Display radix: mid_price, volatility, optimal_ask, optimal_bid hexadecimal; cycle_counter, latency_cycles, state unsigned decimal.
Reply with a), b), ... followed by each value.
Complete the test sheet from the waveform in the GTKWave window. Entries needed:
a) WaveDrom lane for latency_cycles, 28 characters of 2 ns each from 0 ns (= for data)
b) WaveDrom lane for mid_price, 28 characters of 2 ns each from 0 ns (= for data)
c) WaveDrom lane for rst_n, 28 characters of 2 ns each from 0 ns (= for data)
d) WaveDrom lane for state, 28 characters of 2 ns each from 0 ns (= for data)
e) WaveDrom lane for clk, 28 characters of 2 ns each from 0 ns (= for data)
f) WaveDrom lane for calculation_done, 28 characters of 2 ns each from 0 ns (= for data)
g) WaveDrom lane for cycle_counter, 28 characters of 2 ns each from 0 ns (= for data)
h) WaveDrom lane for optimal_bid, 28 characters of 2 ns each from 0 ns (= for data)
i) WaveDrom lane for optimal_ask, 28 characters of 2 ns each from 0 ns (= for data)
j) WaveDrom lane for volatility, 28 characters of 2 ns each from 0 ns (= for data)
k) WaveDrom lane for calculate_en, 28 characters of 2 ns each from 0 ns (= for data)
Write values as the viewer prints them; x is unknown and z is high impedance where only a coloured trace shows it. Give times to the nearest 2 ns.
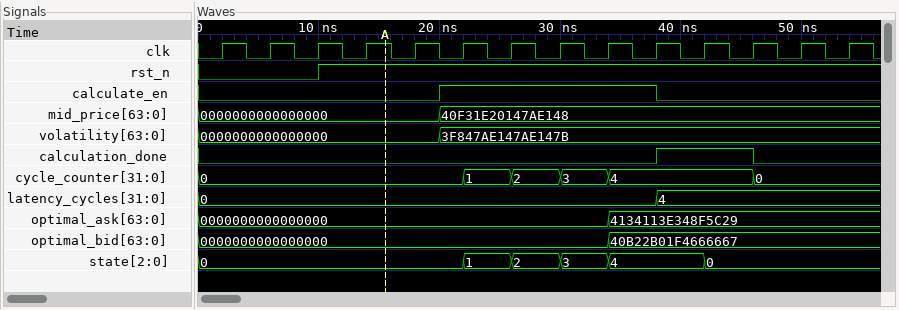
a) {name: 'latency_cycles', wave: '=..................=........', data: '0 4'}
b) {name: 'mid_price', wave: '=.........=.................', data: '0000000000000000 40F31E20147AE148'}
c) {name: 'rst_n', wave: '0....1......................'}
d) {name: 'state', wave: '=..........=.=.=.=...=......', data: '0 1 2 3 4 0'}
e) {name: 'clk', wave: '0101010101010101010101010101'}
f) {name: 'calculation_done', wave: '0..................1...0....'}
g) {name: 'cycle_counter', wave: '=..........=.=.=.=.....=....', data: '0 1 2 3 4 0'}
h) {name: 'optimal_bid', wave: '=................=..........', data: '0000000000000000 40B22B01F4666667'}
i) {name: 'optimal_ask', wave: '=................=..........', data: '0000000000000000 4134113E348F5C29'}
j) {name: 'volatility', wave: '=.........=.................', data: '0000000000000000 3F847AE147AE147B'}
k) {name: 'calculate_en', wave: '0.........1........0........'}
